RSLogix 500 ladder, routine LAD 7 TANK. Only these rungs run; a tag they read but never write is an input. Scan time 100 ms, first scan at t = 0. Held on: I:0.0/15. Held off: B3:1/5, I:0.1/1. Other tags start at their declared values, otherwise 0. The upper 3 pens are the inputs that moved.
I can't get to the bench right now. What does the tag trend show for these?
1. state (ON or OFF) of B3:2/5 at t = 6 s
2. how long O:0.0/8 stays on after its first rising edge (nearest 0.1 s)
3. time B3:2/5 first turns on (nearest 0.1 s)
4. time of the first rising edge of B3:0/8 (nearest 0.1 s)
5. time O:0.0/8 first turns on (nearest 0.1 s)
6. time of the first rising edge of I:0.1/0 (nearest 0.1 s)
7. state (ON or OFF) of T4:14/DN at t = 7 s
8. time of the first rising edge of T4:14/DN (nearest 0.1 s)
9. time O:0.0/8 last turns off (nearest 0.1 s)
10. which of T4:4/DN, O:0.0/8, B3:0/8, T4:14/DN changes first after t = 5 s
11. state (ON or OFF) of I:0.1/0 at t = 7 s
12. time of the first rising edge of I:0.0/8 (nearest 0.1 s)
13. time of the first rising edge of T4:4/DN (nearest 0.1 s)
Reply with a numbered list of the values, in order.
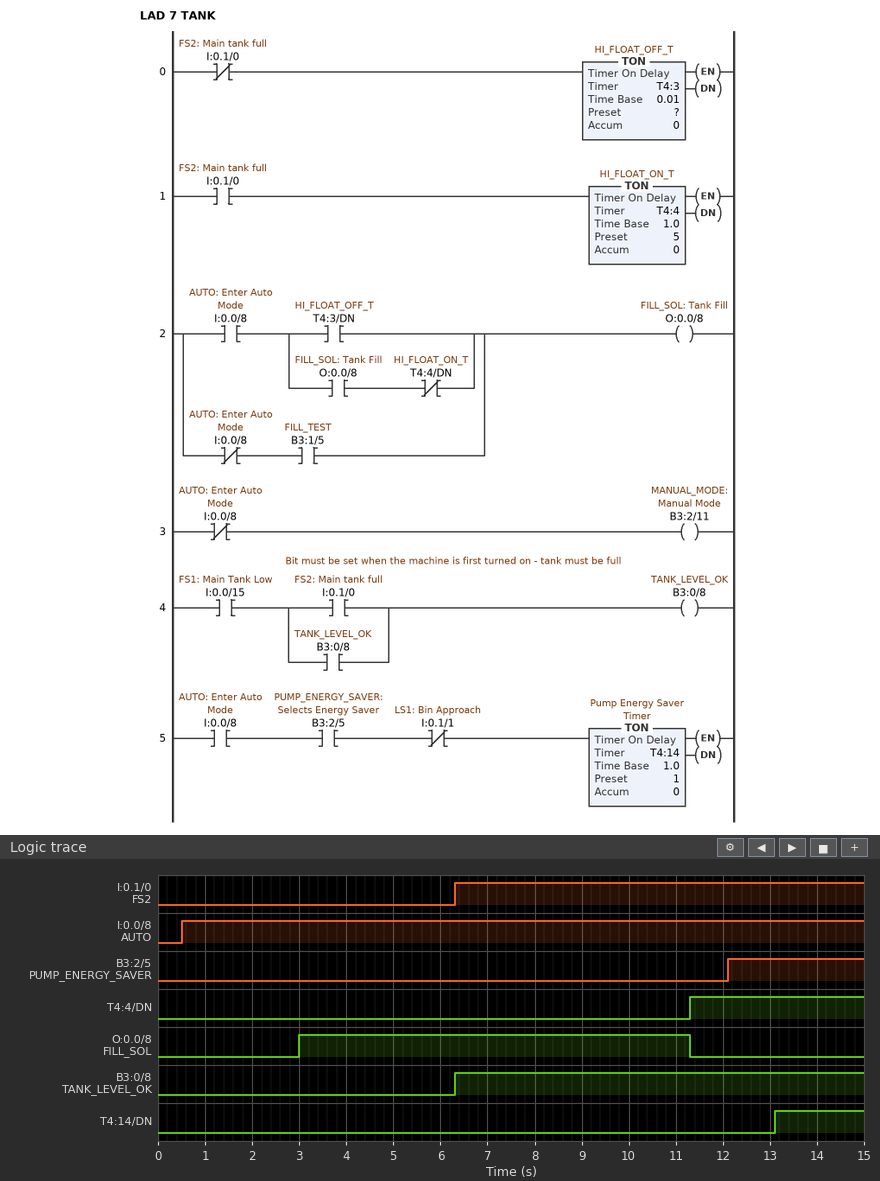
1. OFF
2. 8.3 s
3. 12.1 s
4. 6.3 s
5. 3.0 s
6. 6.3 s
7. OFF
8. 13.1 s
9. 11.3 s
10. B3:0/8
11. ON
12. 0.5 s
13. 11.3 s
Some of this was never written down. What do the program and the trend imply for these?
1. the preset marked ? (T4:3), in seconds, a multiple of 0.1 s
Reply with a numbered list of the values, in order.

1. 3.0 s
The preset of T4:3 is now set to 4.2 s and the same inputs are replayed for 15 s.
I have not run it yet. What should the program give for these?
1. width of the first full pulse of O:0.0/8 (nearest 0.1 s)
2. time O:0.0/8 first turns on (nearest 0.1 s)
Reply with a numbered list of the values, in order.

1. 7.1 s
2. 4.2 s
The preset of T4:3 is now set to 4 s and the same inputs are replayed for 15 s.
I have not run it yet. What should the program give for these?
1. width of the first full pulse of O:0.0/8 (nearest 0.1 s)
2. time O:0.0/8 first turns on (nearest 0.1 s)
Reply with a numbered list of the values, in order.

1. 7.3 s
2. 4.0 s
